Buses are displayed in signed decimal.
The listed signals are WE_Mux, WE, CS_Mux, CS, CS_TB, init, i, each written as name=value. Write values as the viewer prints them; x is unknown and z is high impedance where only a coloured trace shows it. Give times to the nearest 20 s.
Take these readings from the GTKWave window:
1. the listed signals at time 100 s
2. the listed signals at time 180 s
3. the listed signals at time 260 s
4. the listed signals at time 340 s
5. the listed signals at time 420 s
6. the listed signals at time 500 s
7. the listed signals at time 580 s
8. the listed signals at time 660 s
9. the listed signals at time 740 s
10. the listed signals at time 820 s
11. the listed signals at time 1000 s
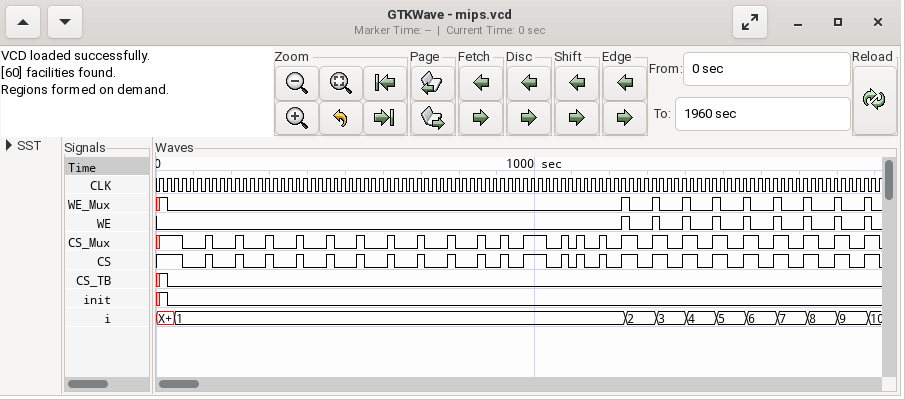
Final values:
WE_Mux=0, WE=0, CS_Mux=0, CS=0, CS_TB=0, init=0, i=1
WE_Mux=0, WE=0, CS_Mux=0, CS=0, CS_TB=0, init=0, i=1
WE_Mux=0, WE=0, CS_Mux=0, CS=0, CS_TB=0, init=0, i=1
WE_Mux=0, WE=0, CS_Mux=0, CS=0, CS_TB=0, init=0, i=1
WE_Mux=0, WE=0, CS_Mux=0, CS=0, CS_TB=0, init=0, i=1
WE_Mux=0, WE=0, CS_Mux=0, CS=0, CS_TB=0, init=0, i=1
WE_Mux=0, WE=0, CS_Mux=0, CS=0, CS_TB=0, init=0, i=1
WE_Mux=0, WE=0, CS_Mux=0, CS=0, CS_TB=0, init=0, i=1
WE_Mux=0, WE=0, CS_Mux=0, CS=0, CS_TB=0, init=0, i=1
WE_Mux=0, WE=0, CS_Mux=0, CS=0, CS_TB=0, init=0, i=1
WE_Mux=0, WE=0, CS_Mux=1, CS=1, CS_TB=0, init=0, i=1
